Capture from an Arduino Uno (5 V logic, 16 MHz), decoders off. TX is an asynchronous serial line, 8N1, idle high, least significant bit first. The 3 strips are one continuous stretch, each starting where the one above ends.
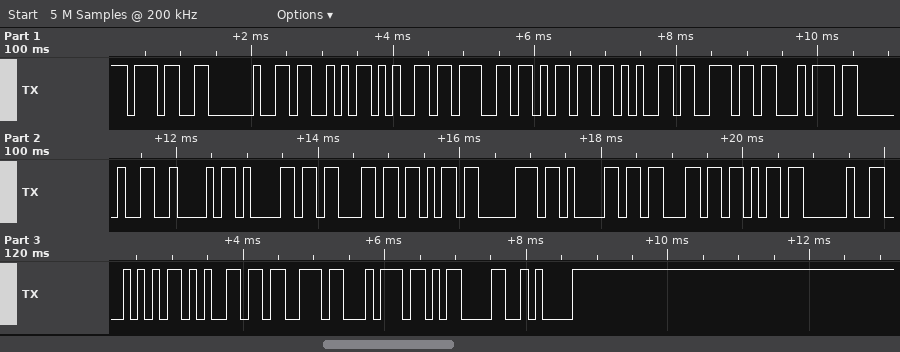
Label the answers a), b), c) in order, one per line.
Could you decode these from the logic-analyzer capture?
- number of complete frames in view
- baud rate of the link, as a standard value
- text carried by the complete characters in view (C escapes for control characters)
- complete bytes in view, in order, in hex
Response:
a) 25
b) 9600 baud
c) "7 Segment Backpack Test\r\n"
d) 37 20 53 65 67 6D 65 6E 74 20 42 61 63 6B 70 61 63 6B 20 54 65 73 74 0D 0A
